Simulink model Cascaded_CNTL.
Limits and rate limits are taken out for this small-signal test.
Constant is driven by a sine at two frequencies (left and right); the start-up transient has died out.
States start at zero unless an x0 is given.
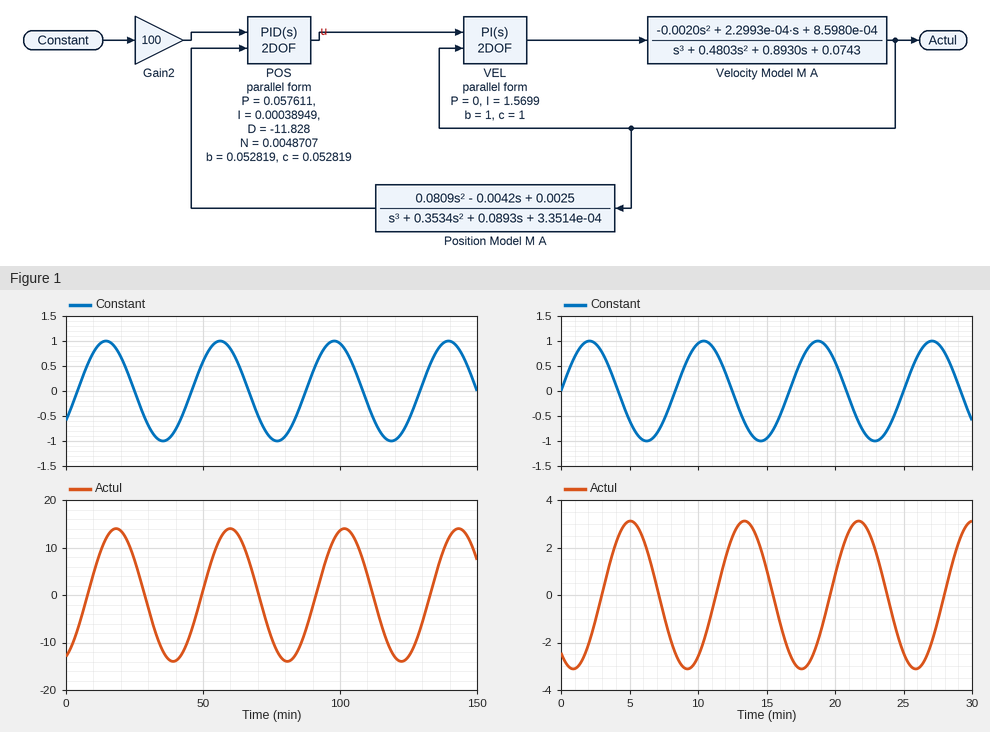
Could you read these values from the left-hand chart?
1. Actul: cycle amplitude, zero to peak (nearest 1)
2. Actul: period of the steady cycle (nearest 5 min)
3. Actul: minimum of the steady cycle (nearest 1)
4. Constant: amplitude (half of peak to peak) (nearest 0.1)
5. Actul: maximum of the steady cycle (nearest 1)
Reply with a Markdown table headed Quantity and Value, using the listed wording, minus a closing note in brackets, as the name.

| Quantity | Value |
|---|---|
| Actul: cycle amplitude, zero to peak | 14 |
| Actul: period of the steady cycle | 40 min |
| Actul: minimum of the steady cycle | -14 |
| Constant: amplitude (half of peak to peak) | 1.0 |
| Actul: maximum of the steady cycle | 14 |
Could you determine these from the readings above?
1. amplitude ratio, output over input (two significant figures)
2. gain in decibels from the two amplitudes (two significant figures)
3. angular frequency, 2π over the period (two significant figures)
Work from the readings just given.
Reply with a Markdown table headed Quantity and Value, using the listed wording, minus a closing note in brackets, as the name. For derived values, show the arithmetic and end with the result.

| Quantity | Value |
|---|---|
| amplitude ratio, output over input | 14 / 1 = 14 |
| gain in decibels from the two amplitudes | 20 log10(14 / 1) = 23 dB |
| angular frequency, 2π over the period | 2π / 40 = 0.16 rad/min |
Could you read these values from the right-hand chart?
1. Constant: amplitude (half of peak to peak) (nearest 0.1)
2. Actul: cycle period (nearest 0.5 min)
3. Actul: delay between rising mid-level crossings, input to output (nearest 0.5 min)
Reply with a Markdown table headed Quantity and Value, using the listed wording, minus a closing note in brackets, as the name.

| Quantity | Value |
|---|---|
| Constant: amplitude (half of peak to peak) | 1.0 |
| Actul: cycle period | 8.5 min |
| Actul: delay between rising mid-level crossings, input to output | 3.0 min |
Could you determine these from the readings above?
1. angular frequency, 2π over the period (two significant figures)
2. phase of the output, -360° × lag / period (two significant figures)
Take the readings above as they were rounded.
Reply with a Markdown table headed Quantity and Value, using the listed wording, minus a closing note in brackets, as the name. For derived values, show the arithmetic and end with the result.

| Quantity | Value |
|---|---|
| angular frequency, 2π over the period | 2π / 8.5 = 0.74 rad/min |
| phase of the output, -360° × lag / period | -360 × 3 / 8.5 = -130° |
